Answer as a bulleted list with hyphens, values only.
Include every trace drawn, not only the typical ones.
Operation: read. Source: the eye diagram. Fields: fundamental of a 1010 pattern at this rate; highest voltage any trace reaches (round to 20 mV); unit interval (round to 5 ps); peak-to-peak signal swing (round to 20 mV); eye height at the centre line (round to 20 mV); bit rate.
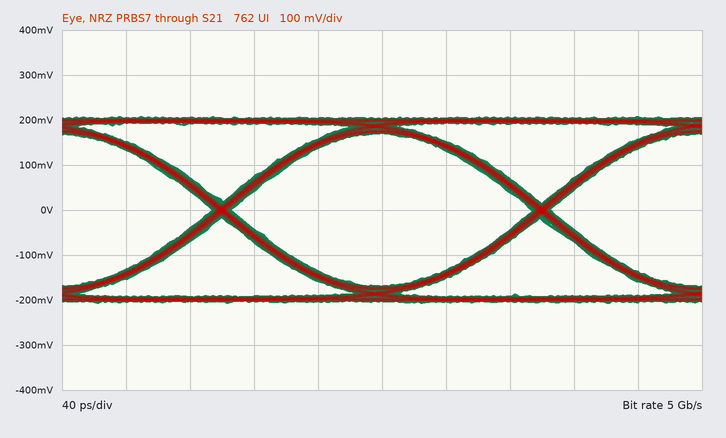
- 2.5 GHz
- 200 mV
- 200 ps
- 420 mV
- 340 mV
- 5 Gb/s
